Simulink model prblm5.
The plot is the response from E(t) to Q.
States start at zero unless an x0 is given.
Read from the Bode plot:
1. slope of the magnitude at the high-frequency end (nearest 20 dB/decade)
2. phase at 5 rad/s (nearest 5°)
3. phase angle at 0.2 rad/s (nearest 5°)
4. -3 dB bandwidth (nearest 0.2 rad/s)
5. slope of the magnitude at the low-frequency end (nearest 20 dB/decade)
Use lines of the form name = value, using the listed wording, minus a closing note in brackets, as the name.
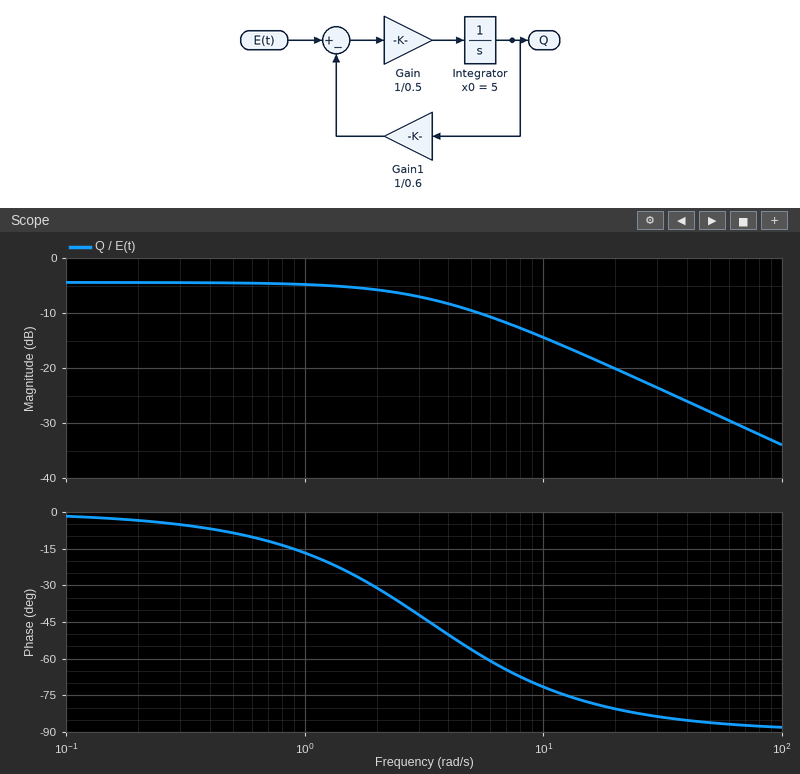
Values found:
slope of the magnitude at the high-frequency end = -20 dB/decade
phase at 5 rad/s = -55°
phase angle at 0.2 rad/s = -5°
-3 dB bandwidth = 3.4 rad/s
slope of the magnitude at the low-frequency end = 0 dB/decade
